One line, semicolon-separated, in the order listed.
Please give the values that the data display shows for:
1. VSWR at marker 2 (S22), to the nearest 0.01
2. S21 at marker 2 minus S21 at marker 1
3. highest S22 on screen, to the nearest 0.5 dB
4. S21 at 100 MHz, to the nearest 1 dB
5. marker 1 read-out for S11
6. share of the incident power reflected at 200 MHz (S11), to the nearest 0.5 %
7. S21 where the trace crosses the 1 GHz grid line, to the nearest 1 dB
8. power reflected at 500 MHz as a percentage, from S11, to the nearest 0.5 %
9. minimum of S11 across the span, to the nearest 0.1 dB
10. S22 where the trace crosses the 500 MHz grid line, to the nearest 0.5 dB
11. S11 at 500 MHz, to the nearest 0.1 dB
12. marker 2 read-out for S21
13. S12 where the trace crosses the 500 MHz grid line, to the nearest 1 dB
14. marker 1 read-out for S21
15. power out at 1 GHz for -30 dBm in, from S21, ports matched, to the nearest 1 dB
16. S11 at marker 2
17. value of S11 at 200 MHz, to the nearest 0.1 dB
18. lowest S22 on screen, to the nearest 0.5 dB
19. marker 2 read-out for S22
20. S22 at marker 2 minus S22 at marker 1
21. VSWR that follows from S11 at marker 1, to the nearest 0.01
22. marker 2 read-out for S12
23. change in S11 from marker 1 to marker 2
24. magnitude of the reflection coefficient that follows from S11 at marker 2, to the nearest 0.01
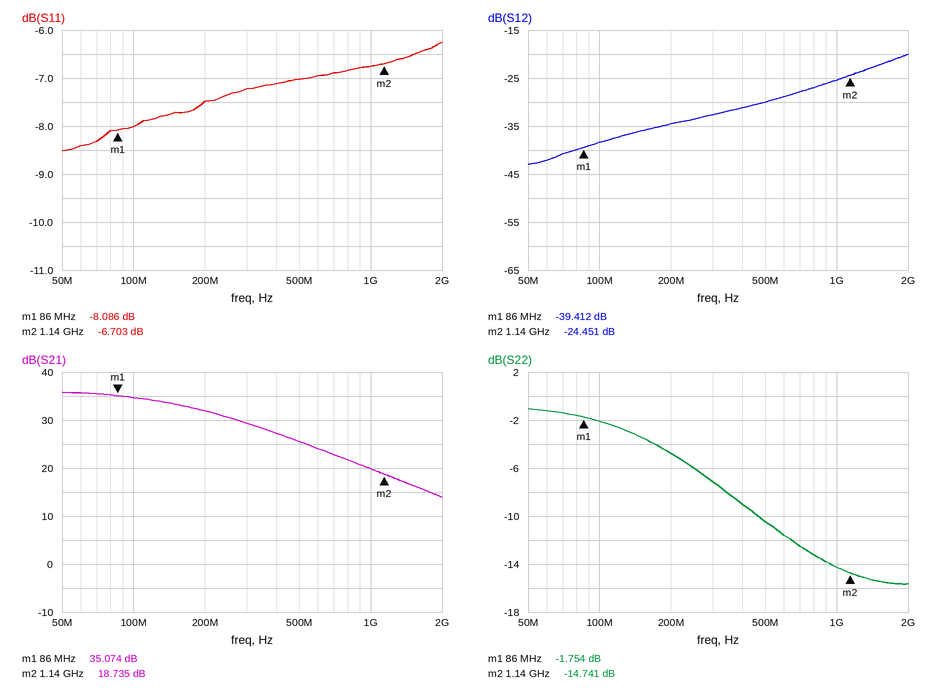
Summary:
1.45; -16.339 dB; -1.0 dB; 35 dB; -8.086 dB; 18.0 %; 20 dB; 20.0 %; -8.5 dB; -10.5 dB; -7.0 dB; 18.735 dB; -30 dB; 35.074 dB; -10 dBm; -6.703 dB; -7.5 dB; -15.5 dB; -14.741 dB; -12.987 dB; 2.30; -24.451 dB; 1.383 dB; 0.46
